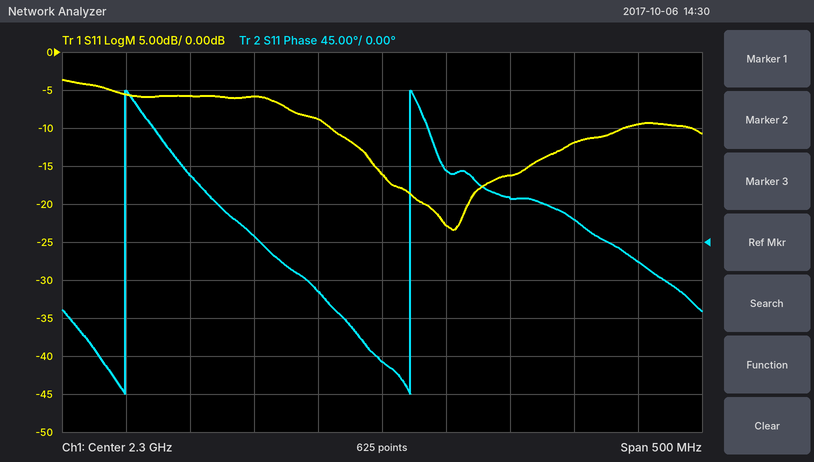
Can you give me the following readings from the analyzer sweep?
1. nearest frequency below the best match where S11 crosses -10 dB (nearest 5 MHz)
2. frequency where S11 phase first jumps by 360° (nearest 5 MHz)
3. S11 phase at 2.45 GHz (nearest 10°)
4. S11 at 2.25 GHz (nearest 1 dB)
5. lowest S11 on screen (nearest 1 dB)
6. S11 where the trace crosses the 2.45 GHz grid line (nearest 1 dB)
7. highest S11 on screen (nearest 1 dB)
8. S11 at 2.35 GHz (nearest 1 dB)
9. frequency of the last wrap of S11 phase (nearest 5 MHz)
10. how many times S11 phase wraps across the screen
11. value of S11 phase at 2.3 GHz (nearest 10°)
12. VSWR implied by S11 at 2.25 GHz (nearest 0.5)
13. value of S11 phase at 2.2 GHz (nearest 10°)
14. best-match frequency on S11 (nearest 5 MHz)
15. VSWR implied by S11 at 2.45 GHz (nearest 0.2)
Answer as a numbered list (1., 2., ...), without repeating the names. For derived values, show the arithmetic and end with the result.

1. 2.260 GHz
2. 2.100 GHz
3. 30°
4. -9 dB
5. -23 dB
6. -12 dB
7. -4 dB
8. -23 dB
9. 2.320 GHz
10. 2
11. -140°
12. |Γ| = 10^(-9/20) = 0.3548; VSWR = (1 + 0.3548)/(1 − 0.3548) ≈ 2.10, so 2.0 to the nearest 0.5
13. 10°
14. 2.355 GHz
15. |Γ| = 10^(-12/20) = 0.2512; VSWR = (1 + 0.2512)/(1 − 0.2512) ≈ 1.67, so 1.6 to the nearest 0.2
